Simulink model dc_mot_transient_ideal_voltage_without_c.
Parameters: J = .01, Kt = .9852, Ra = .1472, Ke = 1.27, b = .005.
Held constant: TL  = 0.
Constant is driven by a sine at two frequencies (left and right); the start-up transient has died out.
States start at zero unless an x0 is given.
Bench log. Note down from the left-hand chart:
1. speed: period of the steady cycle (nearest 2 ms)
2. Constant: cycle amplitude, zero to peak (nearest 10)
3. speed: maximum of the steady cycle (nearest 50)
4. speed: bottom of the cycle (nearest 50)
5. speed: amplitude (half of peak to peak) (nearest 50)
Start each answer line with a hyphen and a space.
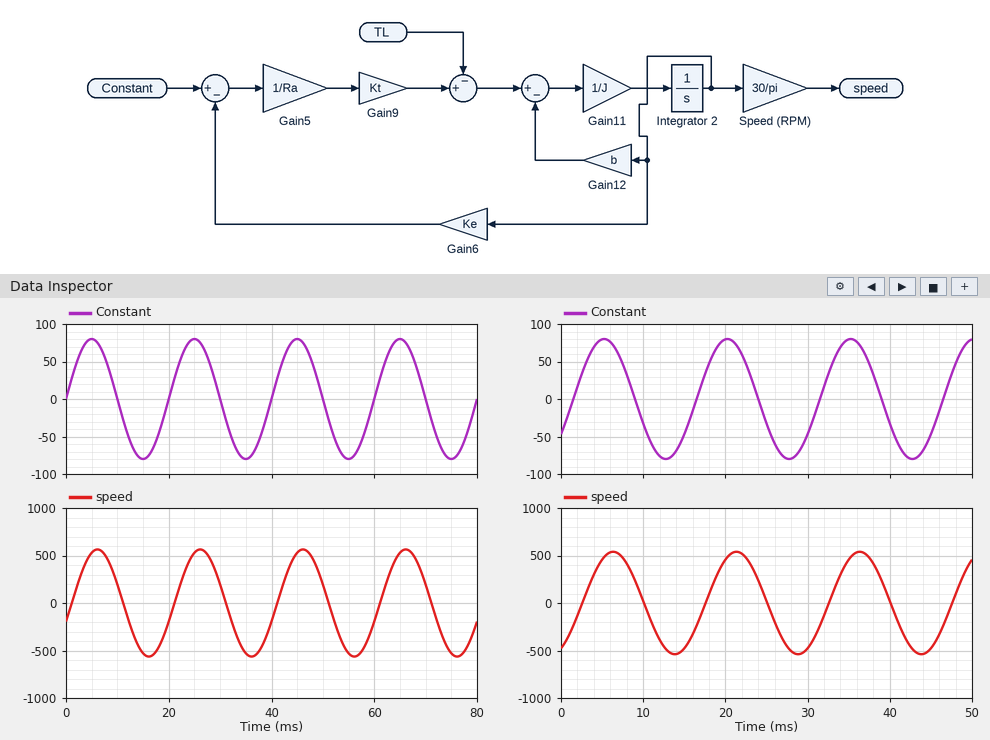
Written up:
- 20 ms
- 80
- 550
- -550
- 550
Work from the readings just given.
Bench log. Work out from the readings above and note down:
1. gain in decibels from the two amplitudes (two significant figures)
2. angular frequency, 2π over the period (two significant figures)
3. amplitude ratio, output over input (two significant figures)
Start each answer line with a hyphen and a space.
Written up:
- 17 dB
- 0.31 rad/ms
- 6.9
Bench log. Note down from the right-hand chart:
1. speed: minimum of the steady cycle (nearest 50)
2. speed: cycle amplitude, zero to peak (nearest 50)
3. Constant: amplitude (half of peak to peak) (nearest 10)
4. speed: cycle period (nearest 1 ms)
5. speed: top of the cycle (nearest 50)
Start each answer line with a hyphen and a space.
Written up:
- -550
- 550
- 80
- 15 ms
- 550
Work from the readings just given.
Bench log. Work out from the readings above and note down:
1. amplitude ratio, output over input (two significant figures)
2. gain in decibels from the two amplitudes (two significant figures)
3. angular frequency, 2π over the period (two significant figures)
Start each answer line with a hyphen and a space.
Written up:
- 6.9
- 17 dB
- 0.42 rad/ms
